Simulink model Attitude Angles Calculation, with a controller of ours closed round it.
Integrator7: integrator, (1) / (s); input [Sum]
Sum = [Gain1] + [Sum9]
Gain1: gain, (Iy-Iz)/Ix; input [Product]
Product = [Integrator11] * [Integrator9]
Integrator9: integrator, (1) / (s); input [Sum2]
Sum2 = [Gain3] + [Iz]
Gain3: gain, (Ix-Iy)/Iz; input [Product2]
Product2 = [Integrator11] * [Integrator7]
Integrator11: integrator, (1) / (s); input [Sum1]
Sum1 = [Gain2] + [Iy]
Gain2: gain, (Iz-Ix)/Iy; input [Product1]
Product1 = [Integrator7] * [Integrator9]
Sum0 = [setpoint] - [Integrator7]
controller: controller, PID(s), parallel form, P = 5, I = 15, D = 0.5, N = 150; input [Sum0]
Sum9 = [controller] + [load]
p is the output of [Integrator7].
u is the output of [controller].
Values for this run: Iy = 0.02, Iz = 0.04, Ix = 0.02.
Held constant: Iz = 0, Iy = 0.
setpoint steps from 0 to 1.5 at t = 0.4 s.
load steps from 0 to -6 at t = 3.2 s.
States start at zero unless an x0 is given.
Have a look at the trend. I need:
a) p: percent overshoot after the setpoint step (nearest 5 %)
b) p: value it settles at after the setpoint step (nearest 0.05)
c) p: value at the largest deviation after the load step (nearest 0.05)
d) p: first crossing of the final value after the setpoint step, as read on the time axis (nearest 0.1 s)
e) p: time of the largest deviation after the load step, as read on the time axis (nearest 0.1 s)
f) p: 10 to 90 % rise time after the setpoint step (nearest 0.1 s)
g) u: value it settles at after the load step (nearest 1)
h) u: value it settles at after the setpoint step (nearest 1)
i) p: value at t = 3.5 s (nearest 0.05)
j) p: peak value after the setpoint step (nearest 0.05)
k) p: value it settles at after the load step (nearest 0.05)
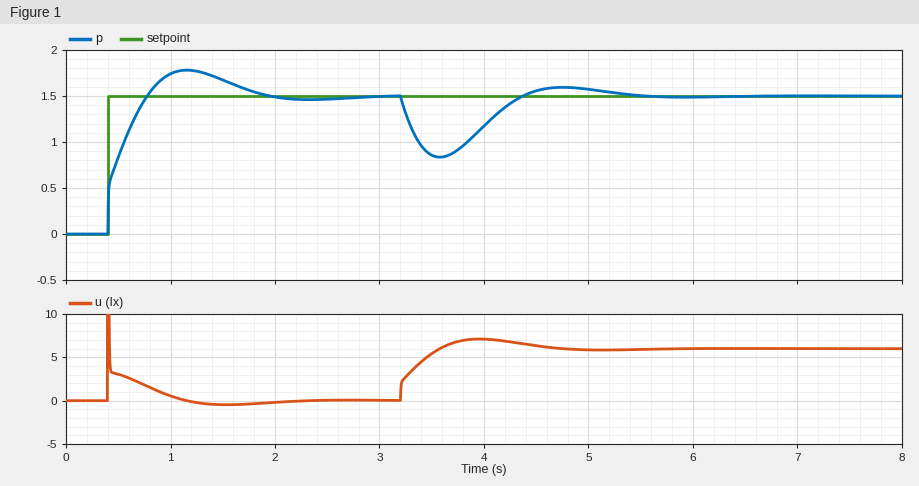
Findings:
20 %
1.50
0.85
0.8 s
3.6 s
0.3 s
6
0
0.85
1.80
1.50
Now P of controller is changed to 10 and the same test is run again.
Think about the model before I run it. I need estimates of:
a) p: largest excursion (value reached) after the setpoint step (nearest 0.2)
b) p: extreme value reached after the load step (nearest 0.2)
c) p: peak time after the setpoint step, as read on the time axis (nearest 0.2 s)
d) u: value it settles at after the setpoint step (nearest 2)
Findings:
1.6
1.0
1.0 s
0
